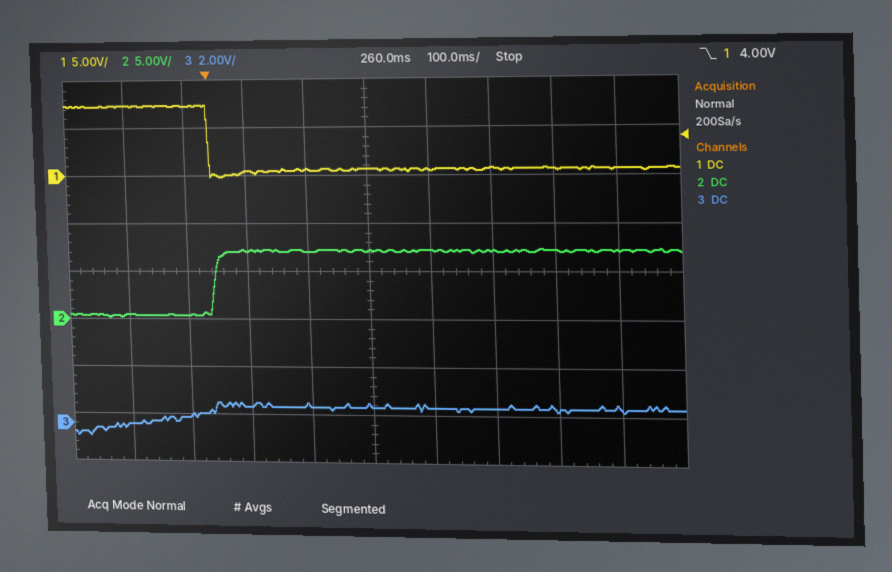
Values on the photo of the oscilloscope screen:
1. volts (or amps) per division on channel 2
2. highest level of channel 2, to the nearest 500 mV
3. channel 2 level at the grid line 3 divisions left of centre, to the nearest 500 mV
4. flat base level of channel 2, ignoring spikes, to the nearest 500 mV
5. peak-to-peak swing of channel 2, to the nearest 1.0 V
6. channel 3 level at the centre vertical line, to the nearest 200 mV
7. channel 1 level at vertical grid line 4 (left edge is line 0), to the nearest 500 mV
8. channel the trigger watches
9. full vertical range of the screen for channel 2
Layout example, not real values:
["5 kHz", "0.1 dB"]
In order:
["5 V", "7.5 V", "500 mV", "500 mV", "7.0 V", "800 mV", "500 mV", "channel 1", "40 V"]
